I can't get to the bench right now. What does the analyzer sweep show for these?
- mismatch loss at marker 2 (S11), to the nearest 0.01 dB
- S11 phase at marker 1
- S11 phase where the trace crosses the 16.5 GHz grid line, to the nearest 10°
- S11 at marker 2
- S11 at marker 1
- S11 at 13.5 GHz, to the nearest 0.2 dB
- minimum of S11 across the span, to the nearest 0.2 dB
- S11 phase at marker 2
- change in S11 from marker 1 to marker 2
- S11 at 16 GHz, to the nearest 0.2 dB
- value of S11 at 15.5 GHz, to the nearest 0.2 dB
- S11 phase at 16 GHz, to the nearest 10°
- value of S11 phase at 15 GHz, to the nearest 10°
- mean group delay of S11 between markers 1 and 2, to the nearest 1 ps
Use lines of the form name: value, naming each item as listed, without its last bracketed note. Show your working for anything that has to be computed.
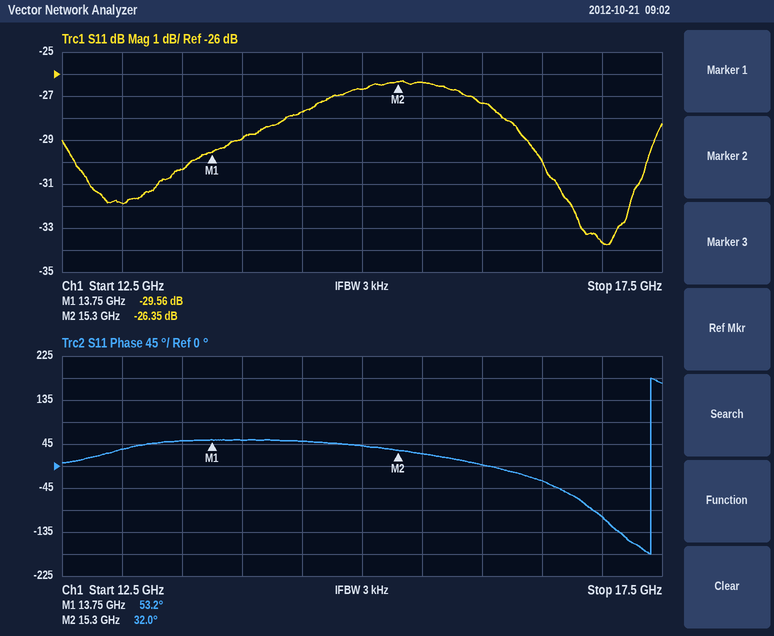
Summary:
mismatch loss at marker 2 (S11), to the nearest 0.01 dB: −10 log10(1 − 10^(-26.35/10)) ≈ 0.01 dB
S11 phase at marker 1: 53.2°
S11 phase where the trace crosses the 16.5 GHz grid line, to the nearest 10°: -30°
S11 at marker 2: -26.35 dB
S11 at marker 1: -29.56 dB
S11 at 13.5 GHz, to the nearest 0.2 dB: -30.4 dB
minimum of S11 across the span, to the nearest 0.2 dB: -33.8 dB
S11 phase at marker 2: 32.0°
change in S11 from marker 1 to marker 2: -26.35 − (-29.56) = 3.21 dB
S11 at 16 GHz, to the nearest 0.2 dB: -27.4 dB
value of S11 at 15.5 GHz, to the nearest 0.2 dB: -26.4 dB
S11 phase at 16 GHz, to the nearest 10°: 0°
value of S11 phase at 15 GHz, to the nearest 10°: 40°
mean group delay of S11 between markers 1 and 2, to the nearest 1 ps: −(32° − (53.2°))/(360° × 1.55 GHz) ≈ 38 ps
